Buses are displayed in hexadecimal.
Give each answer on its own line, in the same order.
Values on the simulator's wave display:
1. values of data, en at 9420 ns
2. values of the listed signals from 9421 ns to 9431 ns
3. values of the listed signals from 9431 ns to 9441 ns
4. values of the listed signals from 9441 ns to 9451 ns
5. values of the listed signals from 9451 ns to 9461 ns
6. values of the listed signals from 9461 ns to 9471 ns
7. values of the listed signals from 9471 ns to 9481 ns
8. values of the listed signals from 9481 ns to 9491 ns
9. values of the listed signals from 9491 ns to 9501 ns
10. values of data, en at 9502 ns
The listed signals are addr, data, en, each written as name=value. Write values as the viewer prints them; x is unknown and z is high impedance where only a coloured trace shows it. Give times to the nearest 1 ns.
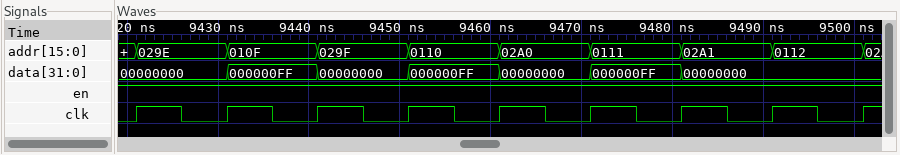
data=00000000, en=1
addr=029E, data=00000000, en=1
addr=010F, data=000000FF, en=1
addr=029F, data=00000000, en=1
addr=0110, data=000000FF, en=1
addr=02A0, data=00000000, en=1
addr=0111, data=000000FF, en=1
addr=02A1, data=00000000, en=1
addr=0112, data=00000000, en=1
data=00000000, en=1
